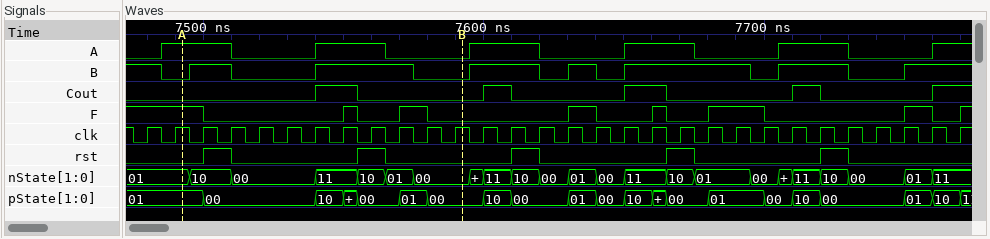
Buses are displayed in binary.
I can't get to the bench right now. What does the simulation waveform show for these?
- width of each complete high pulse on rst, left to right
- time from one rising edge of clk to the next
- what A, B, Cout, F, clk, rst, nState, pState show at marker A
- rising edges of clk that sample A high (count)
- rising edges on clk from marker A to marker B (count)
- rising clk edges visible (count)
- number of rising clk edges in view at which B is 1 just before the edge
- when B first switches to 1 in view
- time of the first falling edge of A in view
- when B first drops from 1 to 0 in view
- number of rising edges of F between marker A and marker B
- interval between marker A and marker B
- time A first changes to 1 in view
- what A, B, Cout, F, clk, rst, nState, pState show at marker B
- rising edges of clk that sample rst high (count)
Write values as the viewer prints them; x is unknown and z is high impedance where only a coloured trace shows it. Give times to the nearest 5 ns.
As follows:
10 ns, 10 ns, 10 ns, 10 ns, 10 ns
10 ns
A=1, B=0, Cout=0, F=1, clk=1, rst=0, nState=01, pState=01
14
10
30
19
7495 ns
7510 ns
7485 ns
2
100 ns
7485 ns
A=0, B=0, Cout=0, F=0, clk=1, rst=0, nState=00, pState=00
5
